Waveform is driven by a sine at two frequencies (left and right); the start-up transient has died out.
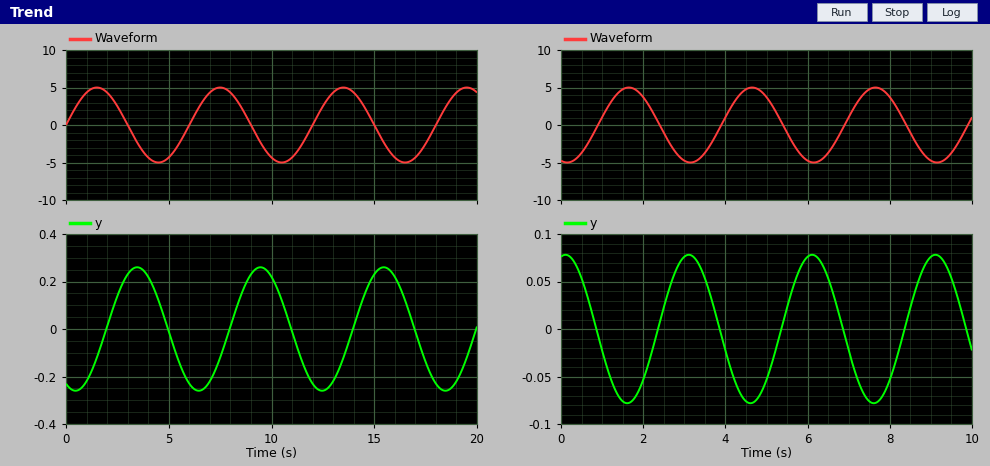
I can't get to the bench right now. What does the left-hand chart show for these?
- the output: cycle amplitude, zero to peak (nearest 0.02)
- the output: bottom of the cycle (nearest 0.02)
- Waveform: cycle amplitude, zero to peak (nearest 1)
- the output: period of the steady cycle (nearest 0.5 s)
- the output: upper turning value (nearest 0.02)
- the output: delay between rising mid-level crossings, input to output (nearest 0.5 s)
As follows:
0.26
-0.26
5
6.0 s
0.26
2.0 s
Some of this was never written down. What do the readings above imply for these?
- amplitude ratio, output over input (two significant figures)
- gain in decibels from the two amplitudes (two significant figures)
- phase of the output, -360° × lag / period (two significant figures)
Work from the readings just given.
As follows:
0.052
-26 dB
-120°
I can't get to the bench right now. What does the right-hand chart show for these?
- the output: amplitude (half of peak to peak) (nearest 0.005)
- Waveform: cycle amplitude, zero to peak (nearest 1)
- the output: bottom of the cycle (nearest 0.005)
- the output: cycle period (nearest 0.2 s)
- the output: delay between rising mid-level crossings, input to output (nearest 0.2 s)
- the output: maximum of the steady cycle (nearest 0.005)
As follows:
0.080
5
-0.080
3.0 s
1.4 s
0.080
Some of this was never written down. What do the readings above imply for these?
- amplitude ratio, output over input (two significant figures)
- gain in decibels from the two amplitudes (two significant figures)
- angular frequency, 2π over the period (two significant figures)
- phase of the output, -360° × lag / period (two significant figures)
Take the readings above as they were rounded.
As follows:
0.016
-36 dB
2.1 rad/s
-170°
